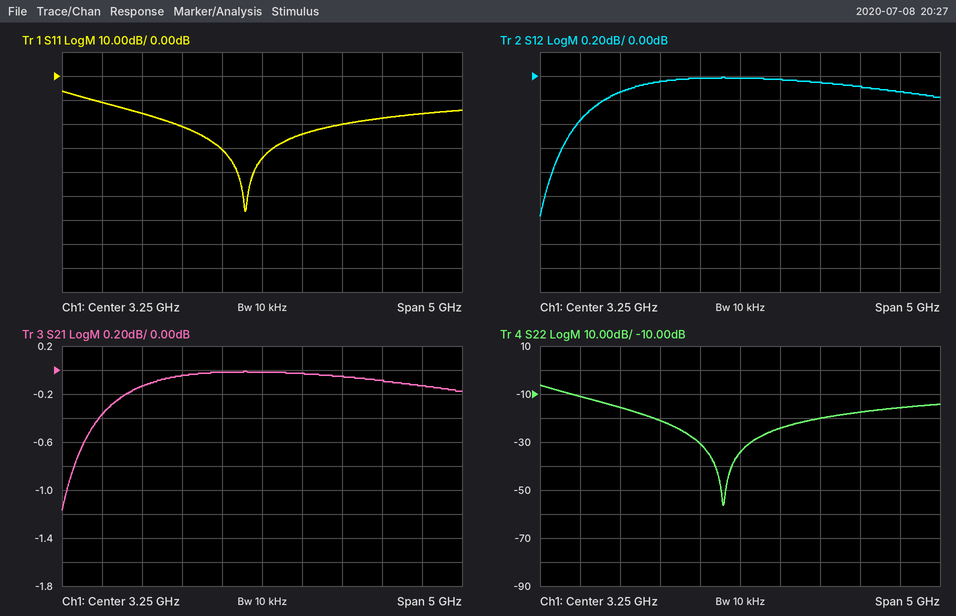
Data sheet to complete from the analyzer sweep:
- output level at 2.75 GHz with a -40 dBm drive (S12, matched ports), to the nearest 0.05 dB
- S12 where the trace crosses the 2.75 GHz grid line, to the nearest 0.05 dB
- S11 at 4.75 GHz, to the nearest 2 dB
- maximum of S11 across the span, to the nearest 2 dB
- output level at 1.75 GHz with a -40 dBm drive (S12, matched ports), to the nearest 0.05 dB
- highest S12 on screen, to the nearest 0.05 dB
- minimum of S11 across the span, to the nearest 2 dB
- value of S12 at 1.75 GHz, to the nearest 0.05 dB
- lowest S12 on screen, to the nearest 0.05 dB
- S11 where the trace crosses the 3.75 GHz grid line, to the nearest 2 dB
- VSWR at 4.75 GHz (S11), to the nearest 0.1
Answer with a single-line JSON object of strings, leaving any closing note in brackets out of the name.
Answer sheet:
{"output level at 2.75 GHz with a -40 dBm drive (S12, matched ports), to the nearest 0.05 dB": "-40.00 dBm", "S12 where the trace crosses the 2.75 GHz grid line, to the nearest 0.05 dB": "0.00 dB", "S11 at 4.75 GHz, to the nearest 2 dB": "-18 dB", "maximum of S11 across the span, to the nearest 2 dB": "-6 dB", "output level at 1.75 GHz with a -40 dBm drive (S12, matched ports), to the nearest 0.05 dB": "-40.15 dBm", "highest S12 on screen, to the nearest 0.05 dB": "0.00 dB", "minimum of S11 across the span, to the nearest 2 dB": "-56 dB", "value of S12 at 1.75 GHz, to the nearest 0.05 dB": "-0.15 dB", "lowest S12 on screen, to the nearest 0.05 dB": "-1.15 dB", "S11 where the trace crosses the 3.75 GHz grid line, to the nearest 2 dB": "-24 dB", "VSWR at 4.75 GHz (S11), to the nearest 0.1": "1.3"}
